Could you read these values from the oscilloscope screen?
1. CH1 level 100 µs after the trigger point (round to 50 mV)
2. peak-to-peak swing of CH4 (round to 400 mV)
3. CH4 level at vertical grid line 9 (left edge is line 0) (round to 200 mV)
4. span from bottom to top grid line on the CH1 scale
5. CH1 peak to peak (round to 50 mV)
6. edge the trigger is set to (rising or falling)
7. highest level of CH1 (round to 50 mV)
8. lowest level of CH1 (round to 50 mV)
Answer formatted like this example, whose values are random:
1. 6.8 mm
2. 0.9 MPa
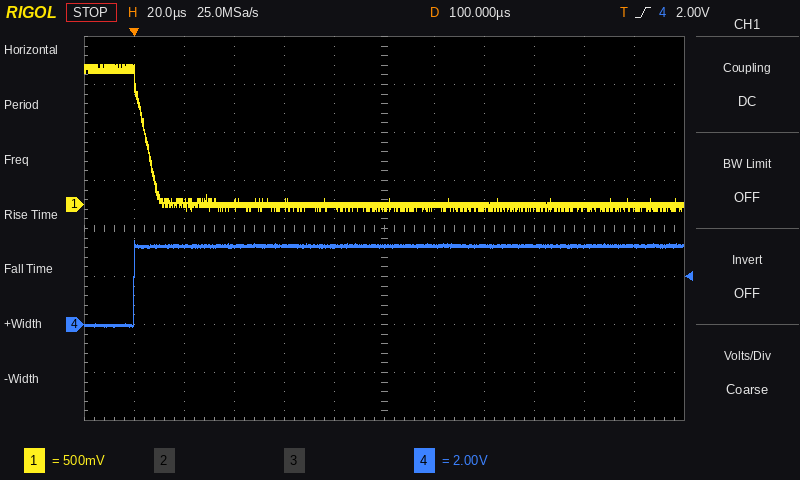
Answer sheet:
1. 0 mV
2. 3.6 V
3. 3.2 V
4. 4 V
5. 1.50 V
6. rising
7. 1.45 V
8. -50 mV
